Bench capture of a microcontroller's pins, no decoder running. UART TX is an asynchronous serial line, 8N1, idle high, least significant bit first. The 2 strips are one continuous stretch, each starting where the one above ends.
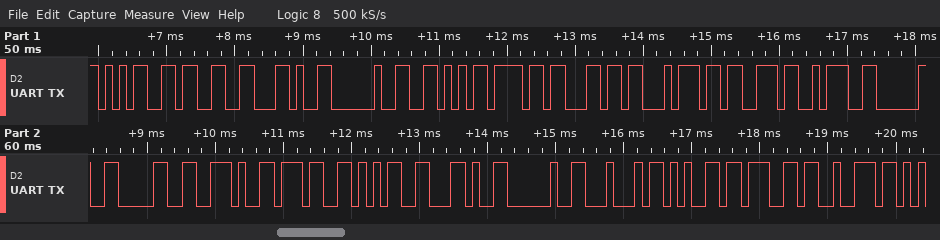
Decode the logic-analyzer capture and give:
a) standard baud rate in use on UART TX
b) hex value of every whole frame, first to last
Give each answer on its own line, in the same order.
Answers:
9600 baud
0x35 0x33 0x2C 0x20 0x56 0x6F 0x6C 0x74 0x73 0x3A 0x20 0x30 0x2E 0x37 0x35 0x2C 0x20 0x44 0x65 0x67 0x72
